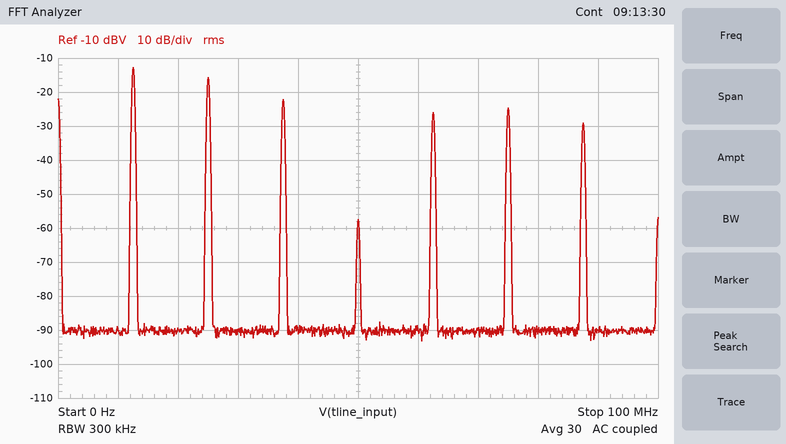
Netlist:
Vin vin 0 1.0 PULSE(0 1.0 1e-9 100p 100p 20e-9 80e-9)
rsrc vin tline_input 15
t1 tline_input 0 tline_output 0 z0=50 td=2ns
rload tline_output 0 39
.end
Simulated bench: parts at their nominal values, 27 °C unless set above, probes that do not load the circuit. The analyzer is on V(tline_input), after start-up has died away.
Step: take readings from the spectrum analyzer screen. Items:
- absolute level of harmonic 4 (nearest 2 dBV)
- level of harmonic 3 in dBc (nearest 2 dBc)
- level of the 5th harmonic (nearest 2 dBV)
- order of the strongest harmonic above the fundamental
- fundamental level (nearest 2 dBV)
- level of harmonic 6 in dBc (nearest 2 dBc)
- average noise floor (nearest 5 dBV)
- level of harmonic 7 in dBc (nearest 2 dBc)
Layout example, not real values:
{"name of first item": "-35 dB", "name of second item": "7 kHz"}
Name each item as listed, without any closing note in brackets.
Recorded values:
{"absolute level of harmonic 4": "-58 dBV", "level of harmonic 3 in dBc": "-10 dBc", "level of the 5th harmonic": "-26 dBV", "order of the strongest harmonic above the fundamental": "2", "fundamental level": "-12 dBV", "level of harmonic 6 in dBc": "-12 dBc", "average noise floor": "-90 dBV", "level of harmonic 7 in dBc": "-16 dBc"}
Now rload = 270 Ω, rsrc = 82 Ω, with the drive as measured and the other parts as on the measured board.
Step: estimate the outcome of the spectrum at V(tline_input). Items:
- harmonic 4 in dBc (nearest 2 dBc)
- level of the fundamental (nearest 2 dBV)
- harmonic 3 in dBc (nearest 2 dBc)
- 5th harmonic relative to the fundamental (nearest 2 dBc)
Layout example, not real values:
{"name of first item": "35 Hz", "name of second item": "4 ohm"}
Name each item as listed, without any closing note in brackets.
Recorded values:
{"harmonic 4 in dBc": "-48 dBc", "level of the fundamental": "-12 dBV", "harmonic 3 in dBc": "-12 dBc", "5th harmonic relative to the fundamental": "-18 dBc"}
